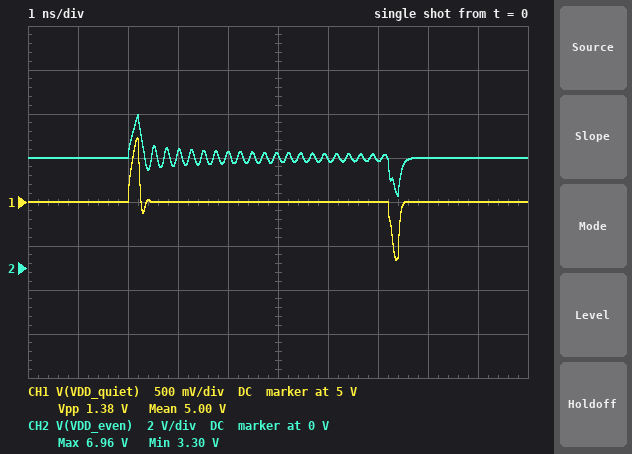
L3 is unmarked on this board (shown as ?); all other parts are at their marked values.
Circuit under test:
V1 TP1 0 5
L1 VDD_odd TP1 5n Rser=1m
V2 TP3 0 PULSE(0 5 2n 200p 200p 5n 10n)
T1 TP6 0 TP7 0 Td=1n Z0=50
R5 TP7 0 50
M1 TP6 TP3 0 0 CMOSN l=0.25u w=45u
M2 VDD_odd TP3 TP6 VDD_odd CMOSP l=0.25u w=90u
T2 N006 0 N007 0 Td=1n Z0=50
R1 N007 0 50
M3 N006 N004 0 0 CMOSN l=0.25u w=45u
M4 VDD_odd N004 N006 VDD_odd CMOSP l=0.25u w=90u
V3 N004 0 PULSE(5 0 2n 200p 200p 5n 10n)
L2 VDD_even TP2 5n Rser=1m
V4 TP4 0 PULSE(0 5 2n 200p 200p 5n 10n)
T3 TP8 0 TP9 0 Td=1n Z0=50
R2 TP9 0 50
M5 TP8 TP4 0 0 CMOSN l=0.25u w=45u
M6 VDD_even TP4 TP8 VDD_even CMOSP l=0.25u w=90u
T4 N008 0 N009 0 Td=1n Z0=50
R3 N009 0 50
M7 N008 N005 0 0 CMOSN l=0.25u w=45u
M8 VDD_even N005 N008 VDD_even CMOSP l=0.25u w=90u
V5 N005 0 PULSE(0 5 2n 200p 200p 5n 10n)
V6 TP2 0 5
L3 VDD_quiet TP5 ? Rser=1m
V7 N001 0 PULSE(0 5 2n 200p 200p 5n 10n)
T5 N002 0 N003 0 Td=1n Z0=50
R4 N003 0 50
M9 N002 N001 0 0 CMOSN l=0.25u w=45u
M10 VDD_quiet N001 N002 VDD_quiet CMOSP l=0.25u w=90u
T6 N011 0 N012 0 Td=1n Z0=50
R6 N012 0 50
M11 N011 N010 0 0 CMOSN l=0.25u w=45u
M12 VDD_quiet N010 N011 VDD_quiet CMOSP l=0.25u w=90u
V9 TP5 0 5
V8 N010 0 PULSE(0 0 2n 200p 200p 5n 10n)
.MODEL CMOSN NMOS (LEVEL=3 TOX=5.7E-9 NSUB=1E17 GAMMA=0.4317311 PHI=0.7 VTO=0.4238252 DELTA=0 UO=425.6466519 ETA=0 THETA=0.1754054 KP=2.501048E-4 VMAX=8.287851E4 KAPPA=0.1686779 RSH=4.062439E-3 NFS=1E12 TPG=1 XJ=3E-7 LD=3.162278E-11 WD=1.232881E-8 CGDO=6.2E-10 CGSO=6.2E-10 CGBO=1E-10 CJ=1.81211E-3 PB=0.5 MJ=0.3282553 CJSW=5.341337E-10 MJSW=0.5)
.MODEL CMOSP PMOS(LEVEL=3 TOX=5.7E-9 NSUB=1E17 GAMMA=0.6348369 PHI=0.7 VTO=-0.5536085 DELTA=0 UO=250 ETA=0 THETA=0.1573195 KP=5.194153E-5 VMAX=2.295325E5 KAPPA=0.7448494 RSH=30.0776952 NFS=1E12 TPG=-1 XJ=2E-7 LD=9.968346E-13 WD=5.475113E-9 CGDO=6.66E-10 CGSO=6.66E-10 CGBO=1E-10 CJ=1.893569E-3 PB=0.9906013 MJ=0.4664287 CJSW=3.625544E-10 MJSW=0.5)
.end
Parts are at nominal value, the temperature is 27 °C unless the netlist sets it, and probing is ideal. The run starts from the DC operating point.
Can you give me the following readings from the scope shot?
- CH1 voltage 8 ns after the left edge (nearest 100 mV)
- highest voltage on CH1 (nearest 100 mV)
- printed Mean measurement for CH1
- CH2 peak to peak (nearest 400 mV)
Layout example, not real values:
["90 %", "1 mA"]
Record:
["5.0 V", "5.7 V", "5.00 V", "3.6 V"]
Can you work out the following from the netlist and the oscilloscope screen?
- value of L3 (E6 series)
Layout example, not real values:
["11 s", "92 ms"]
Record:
["3.3 nH"]
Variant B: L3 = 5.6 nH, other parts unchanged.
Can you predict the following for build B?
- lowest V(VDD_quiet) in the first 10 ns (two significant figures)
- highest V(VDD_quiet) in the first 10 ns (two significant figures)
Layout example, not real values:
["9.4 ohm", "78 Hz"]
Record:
["4.0 V", "6.1 V"]
